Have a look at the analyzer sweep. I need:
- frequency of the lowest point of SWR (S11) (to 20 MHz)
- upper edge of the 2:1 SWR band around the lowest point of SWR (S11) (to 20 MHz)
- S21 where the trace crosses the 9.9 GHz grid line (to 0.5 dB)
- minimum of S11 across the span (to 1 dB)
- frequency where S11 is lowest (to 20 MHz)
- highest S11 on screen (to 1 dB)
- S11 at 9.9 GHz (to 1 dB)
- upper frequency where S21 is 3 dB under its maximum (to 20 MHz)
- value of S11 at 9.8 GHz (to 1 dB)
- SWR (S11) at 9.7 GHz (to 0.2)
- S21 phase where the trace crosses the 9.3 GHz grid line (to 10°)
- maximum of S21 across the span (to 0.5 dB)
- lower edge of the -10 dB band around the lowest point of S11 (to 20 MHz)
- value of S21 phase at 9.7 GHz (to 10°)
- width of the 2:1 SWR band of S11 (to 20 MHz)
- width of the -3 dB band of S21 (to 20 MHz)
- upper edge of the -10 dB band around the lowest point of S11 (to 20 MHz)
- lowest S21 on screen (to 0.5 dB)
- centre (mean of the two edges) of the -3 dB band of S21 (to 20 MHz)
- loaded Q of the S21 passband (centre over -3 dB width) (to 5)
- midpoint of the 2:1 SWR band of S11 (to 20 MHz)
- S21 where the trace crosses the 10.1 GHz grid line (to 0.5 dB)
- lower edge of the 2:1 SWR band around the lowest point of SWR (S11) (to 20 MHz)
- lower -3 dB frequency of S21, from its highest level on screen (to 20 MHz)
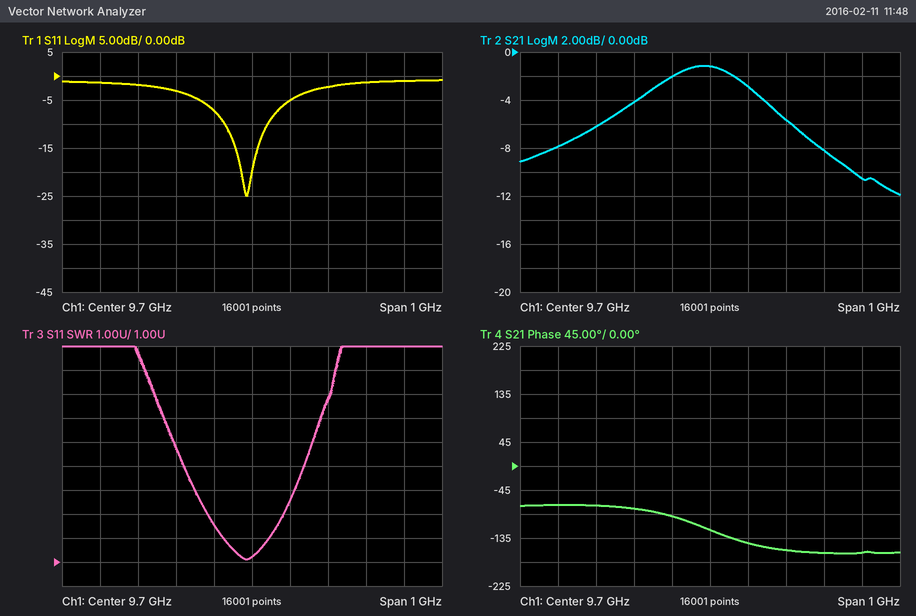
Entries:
9.68 GHz
9.74 GHz
-5.5 dB
-25 dB
9.68 GHz
-1 dB
-2 dB
9.84 GHz
-5 dB
1.2
-70°
-1.0 dB
9.62 GHz
-120°
120 MHz
340 MHz
9.74 GHz
-12.0 dB
9.68 GHz
30
9.68 GHz
-10.5 dB
9.62 GHz
9.50 GHz
